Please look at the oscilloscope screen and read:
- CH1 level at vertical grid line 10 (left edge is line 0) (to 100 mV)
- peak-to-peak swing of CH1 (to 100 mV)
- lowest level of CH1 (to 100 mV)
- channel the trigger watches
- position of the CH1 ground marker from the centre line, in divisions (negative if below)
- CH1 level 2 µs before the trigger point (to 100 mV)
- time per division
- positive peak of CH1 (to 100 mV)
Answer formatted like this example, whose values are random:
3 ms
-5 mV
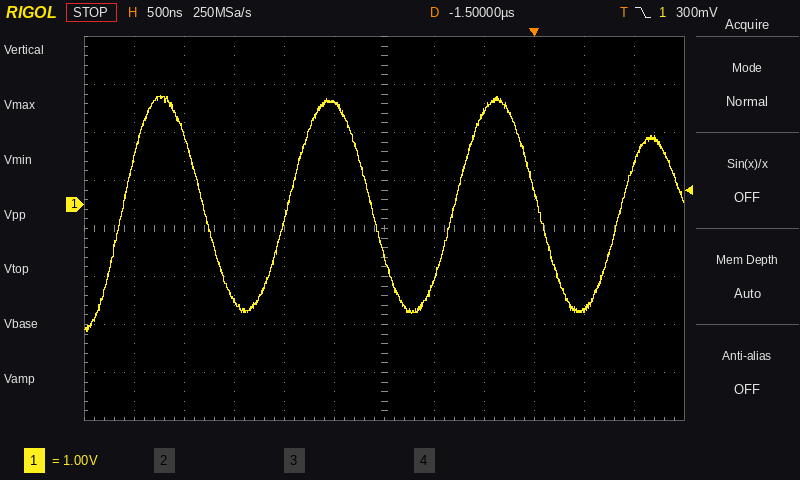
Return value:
-2.2 V
4.9 V
-2.6 V
CH1
+0.5 div
2.1 V
500 ns
2.3 V
